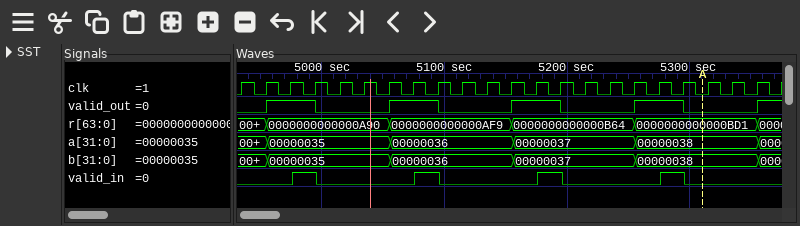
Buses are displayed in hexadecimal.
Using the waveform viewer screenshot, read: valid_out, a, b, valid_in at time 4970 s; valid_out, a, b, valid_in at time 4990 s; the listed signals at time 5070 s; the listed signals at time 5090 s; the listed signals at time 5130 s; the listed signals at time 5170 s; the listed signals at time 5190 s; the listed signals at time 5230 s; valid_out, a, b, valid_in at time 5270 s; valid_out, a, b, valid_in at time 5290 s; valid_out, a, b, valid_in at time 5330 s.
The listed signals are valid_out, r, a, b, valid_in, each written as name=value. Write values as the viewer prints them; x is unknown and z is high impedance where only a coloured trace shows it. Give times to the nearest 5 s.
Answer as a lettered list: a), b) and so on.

a) valid_out=1, a=00000035, b=00000035, valid_in=0
b) valid_out=1, a=00000035, b=00000035, valid_in=1
c) valid_out=1, r=0000000000000AF9, a=00000036, b=00000036, valid_in=0
d) valid_out=1, r=0000000000000AF9, a=00000036, b=00000036, valid_in=1
e) valid_out=0, r=0000000000000AF9, a=00000036, b=00000036, valid_in=0
f) valid_out=1, r=0000000000000B64, a=00000037, b=00000037, valid_in=0
g) valid_out=1, r=0000000000000B64, a=00000037, b=00000037, valid_in=1
h) valid_out=0, r=0000000000000B64, a=00000037, b=00000037, valid_in=0
i) valid_out=1, a=00000038, b=00000038, valid_in=0
j) valid_out=1, a=00000038, b=00000038, valid_in=1
k) valid_out=0, a=00000038, b=00000038, valid_in=0
